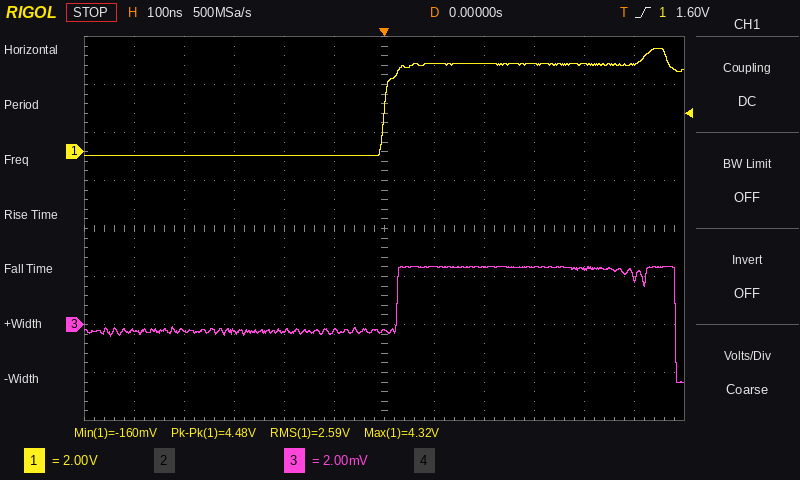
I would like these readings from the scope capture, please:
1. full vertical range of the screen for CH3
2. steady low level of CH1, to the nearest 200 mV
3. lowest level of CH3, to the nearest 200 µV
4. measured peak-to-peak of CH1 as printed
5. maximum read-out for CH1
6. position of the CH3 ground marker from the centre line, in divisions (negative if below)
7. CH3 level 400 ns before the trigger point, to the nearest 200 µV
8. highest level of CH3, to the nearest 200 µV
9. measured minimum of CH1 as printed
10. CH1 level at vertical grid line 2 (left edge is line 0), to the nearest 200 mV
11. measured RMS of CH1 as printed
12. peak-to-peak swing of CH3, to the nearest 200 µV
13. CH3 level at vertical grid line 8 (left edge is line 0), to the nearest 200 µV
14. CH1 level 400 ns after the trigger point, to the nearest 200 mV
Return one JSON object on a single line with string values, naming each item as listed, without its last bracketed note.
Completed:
{"full vertical range of the screen for CH3": "16 mV", "steady low level of CH1, to the nearest 200 mV": "-200 mV", "lowest level of CH3, to the nearest 200 µV": "-2.4 mV", "measured peak-to-peak of CH1 as printed": "4.48 V", "maximum read-out for CH1": "4.32 V", "position of the CH3 ground marker from the centre line, in divisions": "-2.0 div", "CH3 level 400 ns before the trigger point, to the nearest 200 µV": "-200 µV", "highest level of CH3, to the nearest 200 µV": "2.4 mV", "measured minimum of CH1 as printed": "-160 mV", "CH1 level at vertical grid line 2 (left edge is line 0), to the nearest 200 mV": "-200 mV", "measured RMS of CH1 as printed": "2.59 V", "peak-to-peak swing of CH3, to the nearest 200 µV": "4.8 mV", "CH3 level at vertical grid line 8 (left edge is line 0), to the nearest 200 µV": "2.4 mV", "CH1 level 400 ns after the trigger point, to the nearest 200 mV": "3.6 V"}
